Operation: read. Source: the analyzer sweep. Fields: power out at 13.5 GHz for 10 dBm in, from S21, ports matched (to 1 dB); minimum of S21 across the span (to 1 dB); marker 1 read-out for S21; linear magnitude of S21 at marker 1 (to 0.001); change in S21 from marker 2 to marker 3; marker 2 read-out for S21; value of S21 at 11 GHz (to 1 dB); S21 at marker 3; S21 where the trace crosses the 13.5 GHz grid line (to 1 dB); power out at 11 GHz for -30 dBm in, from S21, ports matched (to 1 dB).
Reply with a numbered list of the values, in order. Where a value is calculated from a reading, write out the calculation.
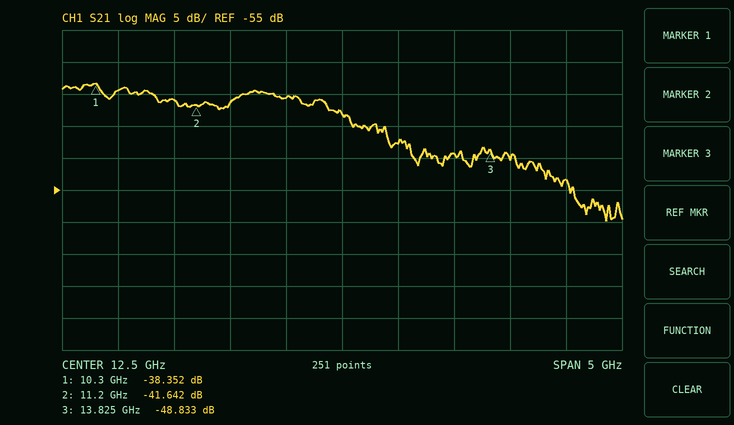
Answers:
1. 10 dBm + (-49 dB) = -39 dBm
2. -60 dB
3. -38.352 dB
4. 10^(-38.352/20) ≈ 0.012
5. -48.833 − (-41.642) = -7.191 dB
6. -41.642 dB
7. -41 dB
8. -48.833 dB
9. -49 dB
10. -30 dBm + (-41 dB) = -71 dBm
